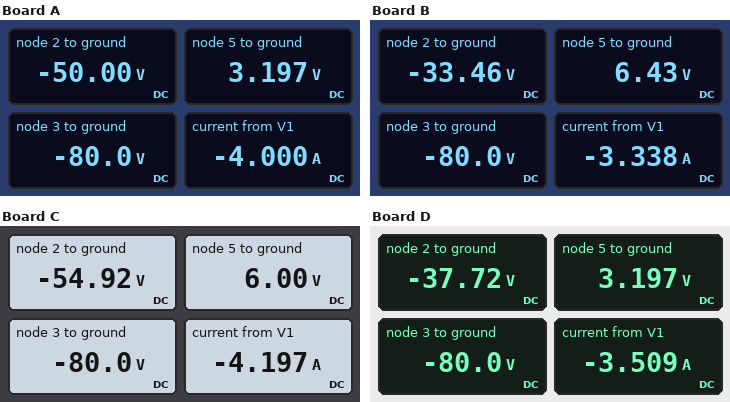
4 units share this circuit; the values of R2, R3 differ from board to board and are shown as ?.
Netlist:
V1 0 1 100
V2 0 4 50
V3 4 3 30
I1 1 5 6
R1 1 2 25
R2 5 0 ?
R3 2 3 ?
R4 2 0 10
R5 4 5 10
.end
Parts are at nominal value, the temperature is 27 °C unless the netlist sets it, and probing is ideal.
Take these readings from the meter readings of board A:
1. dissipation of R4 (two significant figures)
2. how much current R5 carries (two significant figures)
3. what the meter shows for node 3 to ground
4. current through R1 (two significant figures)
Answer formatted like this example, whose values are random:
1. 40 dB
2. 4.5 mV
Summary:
1. 250 W
2. 5.3 A
3. -80.0 V
4. 2.0 A
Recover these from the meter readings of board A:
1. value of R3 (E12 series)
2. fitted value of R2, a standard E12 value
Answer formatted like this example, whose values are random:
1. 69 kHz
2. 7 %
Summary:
1. 10 Ω
2. 4.7 Ω
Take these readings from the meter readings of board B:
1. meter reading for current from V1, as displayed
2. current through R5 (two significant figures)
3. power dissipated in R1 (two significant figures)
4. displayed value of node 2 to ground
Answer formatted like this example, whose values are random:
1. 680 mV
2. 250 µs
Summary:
1. -3.338 A
2. 5.6 A
3. 180 W
4. -33.46 V
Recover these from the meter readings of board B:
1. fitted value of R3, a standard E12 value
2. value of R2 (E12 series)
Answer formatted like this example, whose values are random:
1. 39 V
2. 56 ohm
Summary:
1. 68 Ω
2. 18 Ω
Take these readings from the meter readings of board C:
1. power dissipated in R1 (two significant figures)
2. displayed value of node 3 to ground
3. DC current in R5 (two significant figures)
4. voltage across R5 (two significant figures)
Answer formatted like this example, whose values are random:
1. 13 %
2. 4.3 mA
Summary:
1. 81 W
2. -80.0 V
3. 5.6 A
4. 56 V
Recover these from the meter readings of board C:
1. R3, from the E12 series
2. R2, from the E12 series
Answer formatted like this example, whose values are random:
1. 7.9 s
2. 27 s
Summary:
1. 6.8 Ω
2. 15 Ω
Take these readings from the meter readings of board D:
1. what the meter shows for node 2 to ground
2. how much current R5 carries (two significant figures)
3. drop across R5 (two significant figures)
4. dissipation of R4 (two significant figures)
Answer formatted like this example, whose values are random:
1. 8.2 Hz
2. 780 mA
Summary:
1. -37.72 V
2. 5.3 A
3. 53 V
4. 140 W
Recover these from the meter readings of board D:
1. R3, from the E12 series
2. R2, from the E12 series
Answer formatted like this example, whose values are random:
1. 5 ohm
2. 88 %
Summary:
1. 33 Ω
2. 4.7 Ω
